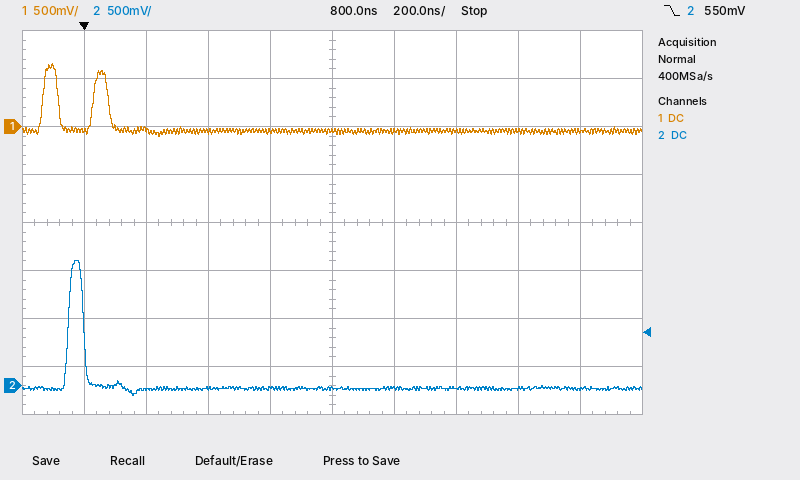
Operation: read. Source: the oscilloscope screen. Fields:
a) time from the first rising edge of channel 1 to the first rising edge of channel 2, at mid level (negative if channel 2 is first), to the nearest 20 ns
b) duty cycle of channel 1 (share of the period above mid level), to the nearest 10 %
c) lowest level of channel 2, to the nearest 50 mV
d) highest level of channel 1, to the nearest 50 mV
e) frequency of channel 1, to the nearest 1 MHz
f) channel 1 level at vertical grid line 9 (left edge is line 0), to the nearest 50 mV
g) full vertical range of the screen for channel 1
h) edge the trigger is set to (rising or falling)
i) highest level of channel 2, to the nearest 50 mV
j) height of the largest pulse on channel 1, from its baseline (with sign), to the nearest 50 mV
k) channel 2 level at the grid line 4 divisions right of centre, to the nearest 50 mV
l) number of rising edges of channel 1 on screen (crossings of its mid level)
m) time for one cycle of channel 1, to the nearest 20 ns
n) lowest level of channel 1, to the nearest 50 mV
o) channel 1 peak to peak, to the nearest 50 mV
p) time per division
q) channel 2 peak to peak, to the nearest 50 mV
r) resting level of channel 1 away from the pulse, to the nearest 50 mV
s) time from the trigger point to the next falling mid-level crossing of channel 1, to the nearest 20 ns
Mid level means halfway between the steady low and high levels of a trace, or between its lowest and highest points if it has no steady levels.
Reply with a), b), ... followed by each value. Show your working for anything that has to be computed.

a) +80 ns
b) 30 %
c) -100 mV
d) 650 mV
e) 1 / 160 ns ≈ 6 MHz
f) -50 mV
g) 4 V
h) falling
i) 1.30 V
j) 650 mV − (-50 mV) = +700 mV
k) -50 mV
l) 2
m) 160 ns
n) -100 mV
o) 650 mV − (-100 mV) = 750 mV
p) 200 ns
q) 1.30 V − (-100 mV) = 1.40 V
r) -50 mV
s) 80 ns
